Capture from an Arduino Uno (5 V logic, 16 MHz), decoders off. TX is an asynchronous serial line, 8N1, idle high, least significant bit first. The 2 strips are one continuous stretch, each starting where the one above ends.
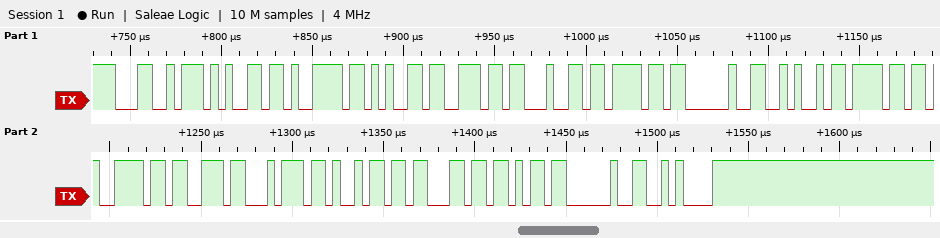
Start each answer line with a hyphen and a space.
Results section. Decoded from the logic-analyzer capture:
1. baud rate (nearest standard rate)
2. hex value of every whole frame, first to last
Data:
- 250000 baud
- 4C 65 79 65 6E 64 6F 20 4A 6F 79 73 74 69 63 6B 20 0A
